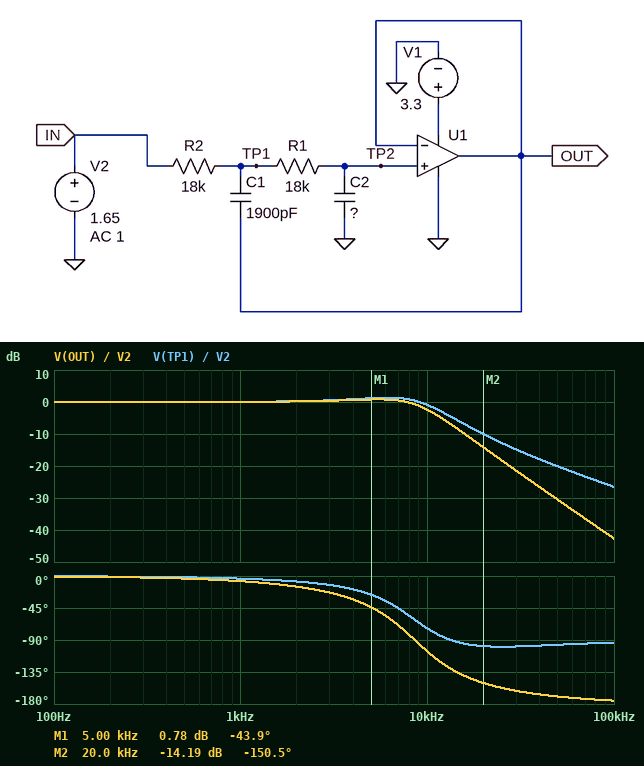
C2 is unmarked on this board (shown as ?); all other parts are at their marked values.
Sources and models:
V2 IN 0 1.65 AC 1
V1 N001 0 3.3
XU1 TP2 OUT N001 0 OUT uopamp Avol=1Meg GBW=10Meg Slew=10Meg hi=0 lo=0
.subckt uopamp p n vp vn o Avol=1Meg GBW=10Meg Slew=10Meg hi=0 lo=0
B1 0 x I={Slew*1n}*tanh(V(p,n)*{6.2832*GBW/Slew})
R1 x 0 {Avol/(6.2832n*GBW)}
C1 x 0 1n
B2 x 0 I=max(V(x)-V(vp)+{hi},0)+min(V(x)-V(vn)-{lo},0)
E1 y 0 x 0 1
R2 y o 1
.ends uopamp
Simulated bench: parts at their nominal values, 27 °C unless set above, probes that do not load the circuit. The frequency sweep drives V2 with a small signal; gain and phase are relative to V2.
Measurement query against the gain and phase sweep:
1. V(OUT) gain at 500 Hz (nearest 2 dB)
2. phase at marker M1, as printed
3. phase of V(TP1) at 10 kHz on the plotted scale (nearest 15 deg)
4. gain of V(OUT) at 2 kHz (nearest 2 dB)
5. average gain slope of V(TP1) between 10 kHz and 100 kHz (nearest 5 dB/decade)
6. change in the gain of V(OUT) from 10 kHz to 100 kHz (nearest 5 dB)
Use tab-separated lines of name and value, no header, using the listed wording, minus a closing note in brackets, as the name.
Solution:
V(OUT) gain at 500 Hz	0 dB
phase at marker M1, as printed	-43.9 deg
phase of V(TP1) at 10 kHz on the plotted scale	-75 deg
gain of V(OUT) at 2 kHz	0 dB
average gain slope of V(TP1) between 10 kHz and 100 kHz	-25 dB/decade
change in the gain of V(OUT) from 10 kHz to 100 kHz	-40 dB
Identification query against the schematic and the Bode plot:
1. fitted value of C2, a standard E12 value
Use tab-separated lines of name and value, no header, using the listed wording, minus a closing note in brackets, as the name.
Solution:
fitted value of C2, a standard E12 value	560 pF
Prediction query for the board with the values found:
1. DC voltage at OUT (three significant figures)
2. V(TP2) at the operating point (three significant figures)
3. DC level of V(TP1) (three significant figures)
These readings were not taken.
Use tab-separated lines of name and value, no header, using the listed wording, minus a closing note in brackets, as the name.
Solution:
DC voltage at OUT	1.65 V
V(TP2) at the operating point	1.65 V
DC level of V(TP1)	1.65 V
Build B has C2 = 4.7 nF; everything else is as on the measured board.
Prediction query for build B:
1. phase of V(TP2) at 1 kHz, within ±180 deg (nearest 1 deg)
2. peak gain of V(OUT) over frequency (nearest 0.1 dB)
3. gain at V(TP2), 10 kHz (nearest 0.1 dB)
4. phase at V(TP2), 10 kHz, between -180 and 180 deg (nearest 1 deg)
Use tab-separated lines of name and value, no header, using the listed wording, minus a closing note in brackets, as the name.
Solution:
phase of V(TP2) at 1 kHz, within ±180 deg	-50 deg
peak gain of V(OUT) over frequency	0 dB
gain at V(TP2), 10 kHz	-23.5 dB
phase at V(TP2), 10 kHz, between -180 and 180 deg	-134 deg
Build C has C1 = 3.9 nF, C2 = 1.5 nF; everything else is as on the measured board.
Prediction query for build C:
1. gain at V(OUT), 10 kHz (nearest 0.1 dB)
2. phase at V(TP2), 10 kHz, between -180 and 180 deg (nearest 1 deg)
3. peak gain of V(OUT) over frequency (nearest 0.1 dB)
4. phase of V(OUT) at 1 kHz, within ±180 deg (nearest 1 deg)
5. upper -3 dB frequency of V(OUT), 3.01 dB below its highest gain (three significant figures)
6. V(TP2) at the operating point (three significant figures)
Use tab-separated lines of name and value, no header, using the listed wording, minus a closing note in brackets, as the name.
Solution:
gain at V(OUT), 10 kHz	-17.3 dB
phase at V(TP2), 10 kHz, between -180 and 180 deg	-152 deg
peak gain of V(OUT) over frequency	0.2 dB
phase of V(OUT) at 1 kHz, within ±180 deg	-20 deg
upper -3 dB frequency of V(OUT), 3.01 dB below its highest gain	4.01 kHz
V(TP2) at the operating point	1.65 V
